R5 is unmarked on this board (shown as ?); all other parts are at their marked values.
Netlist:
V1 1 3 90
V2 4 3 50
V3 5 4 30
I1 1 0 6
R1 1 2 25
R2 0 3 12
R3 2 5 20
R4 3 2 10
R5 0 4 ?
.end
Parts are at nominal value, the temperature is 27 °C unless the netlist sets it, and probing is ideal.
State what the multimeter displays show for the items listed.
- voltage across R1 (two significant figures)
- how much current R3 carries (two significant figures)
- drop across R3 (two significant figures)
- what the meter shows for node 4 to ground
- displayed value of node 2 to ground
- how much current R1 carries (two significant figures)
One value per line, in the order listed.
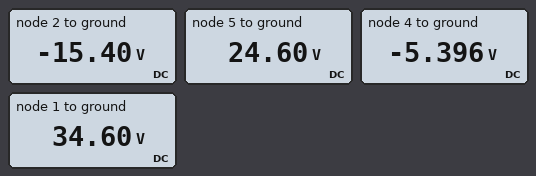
50 V
2.0 A
40 V
-5.396 V
-15.40 V
2.0 A
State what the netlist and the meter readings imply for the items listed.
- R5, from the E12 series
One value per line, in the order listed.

3.9 Ω
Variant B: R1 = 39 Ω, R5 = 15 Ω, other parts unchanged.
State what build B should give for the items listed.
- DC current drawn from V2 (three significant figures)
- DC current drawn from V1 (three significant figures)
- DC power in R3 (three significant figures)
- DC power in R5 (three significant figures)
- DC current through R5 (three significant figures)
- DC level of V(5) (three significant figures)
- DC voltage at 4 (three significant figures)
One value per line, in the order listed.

1.39 A
7.39 A
97.2 W
9.96 W
815 mA
17.8 V
-12.2 V
